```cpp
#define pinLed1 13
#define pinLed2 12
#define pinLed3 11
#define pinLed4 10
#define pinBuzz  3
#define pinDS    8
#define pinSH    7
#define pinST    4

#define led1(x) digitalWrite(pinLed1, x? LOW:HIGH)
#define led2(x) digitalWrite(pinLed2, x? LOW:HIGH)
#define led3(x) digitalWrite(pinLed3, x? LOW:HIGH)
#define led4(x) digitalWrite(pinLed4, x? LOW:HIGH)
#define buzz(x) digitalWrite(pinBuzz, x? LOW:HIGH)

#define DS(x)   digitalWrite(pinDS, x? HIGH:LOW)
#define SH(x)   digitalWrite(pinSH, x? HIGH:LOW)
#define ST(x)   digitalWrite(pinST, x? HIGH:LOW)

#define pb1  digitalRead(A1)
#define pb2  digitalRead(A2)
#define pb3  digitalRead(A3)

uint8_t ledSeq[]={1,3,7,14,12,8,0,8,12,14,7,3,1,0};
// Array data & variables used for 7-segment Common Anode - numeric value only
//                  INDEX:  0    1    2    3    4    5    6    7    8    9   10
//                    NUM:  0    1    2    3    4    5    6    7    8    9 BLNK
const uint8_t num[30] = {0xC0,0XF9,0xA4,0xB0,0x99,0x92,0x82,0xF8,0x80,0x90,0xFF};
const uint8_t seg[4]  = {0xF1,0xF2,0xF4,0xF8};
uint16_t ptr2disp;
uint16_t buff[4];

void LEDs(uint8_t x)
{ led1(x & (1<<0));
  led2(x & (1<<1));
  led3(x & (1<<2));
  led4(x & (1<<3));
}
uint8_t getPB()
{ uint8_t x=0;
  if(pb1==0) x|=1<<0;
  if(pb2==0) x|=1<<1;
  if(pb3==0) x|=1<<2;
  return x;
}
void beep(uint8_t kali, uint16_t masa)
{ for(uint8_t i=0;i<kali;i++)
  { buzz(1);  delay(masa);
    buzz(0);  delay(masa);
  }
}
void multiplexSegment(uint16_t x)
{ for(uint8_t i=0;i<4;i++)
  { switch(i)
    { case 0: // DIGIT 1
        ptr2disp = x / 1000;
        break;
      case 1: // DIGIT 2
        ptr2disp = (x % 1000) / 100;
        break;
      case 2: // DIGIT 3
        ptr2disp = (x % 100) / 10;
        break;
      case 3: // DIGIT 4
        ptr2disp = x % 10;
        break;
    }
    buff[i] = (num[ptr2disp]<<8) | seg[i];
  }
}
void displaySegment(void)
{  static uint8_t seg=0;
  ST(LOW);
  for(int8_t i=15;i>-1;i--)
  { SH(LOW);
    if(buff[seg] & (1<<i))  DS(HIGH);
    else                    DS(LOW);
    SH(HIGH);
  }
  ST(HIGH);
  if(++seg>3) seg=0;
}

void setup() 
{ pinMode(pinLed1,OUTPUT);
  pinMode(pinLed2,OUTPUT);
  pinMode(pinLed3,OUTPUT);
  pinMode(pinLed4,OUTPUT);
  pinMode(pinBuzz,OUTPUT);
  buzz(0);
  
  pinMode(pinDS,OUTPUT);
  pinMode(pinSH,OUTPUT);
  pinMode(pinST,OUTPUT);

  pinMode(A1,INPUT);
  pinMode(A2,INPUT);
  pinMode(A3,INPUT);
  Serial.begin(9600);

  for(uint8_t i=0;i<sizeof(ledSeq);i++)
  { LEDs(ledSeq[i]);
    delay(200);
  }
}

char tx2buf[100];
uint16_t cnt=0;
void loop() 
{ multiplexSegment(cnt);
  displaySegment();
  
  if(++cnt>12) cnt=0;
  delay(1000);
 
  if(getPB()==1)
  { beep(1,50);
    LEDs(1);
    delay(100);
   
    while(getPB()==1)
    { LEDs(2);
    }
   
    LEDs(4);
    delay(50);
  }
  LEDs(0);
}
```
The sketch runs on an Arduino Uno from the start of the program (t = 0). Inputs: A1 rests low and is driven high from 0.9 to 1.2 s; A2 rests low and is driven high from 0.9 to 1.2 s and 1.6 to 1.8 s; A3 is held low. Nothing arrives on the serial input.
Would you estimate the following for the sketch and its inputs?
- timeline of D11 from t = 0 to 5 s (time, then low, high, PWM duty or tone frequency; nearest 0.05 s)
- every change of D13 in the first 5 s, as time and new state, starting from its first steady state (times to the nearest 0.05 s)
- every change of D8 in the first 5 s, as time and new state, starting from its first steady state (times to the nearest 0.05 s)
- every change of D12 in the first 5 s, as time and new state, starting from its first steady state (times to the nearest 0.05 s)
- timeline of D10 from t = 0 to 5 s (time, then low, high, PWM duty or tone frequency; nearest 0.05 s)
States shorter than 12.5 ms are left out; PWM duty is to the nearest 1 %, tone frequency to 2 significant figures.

0 s high; 0.4 s low; 1 s high; 1.6 s low; 2.2 s high
0 s low; 0.6 s high; 2 s low; 2.6 s high
0 s low; 2.8 s high; 3.8 s low
0 s high; 0.2 s low; 0.8 s high; 1.8 s low; 2.4 s high
0 s high; 0.6 s low; 1.2 s high; 1.4 s low; 2 s high
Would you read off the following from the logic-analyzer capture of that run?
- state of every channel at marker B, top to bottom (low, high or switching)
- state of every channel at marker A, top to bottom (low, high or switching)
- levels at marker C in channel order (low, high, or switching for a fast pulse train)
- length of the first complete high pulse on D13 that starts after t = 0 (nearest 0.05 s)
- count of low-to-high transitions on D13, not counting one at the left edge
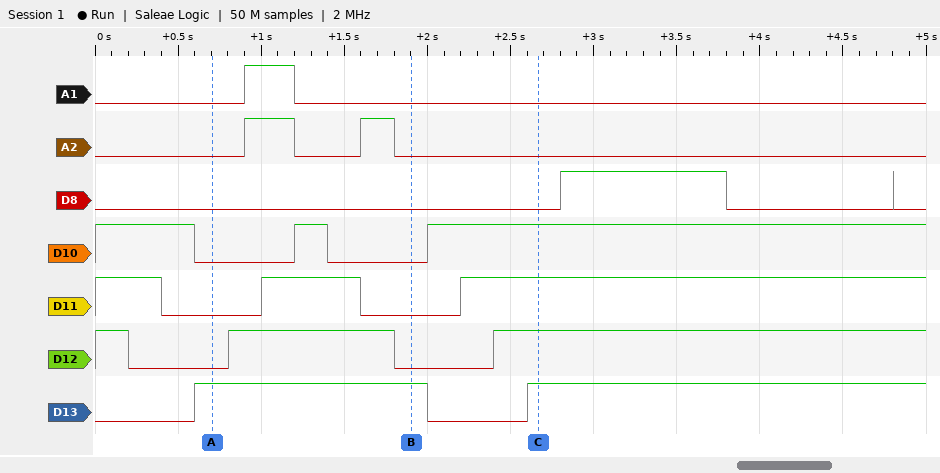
A1 low, A2 low, D8 low, D10 low, D11 low, D12 low, D13 high
A1 low, A2 low, D8 low, D10 low, D11 low, D12 low, D13 high
A1 low, A2 low, D8 low, D10 high, D11 high, D12 high, D13 high
1.40 s
2
